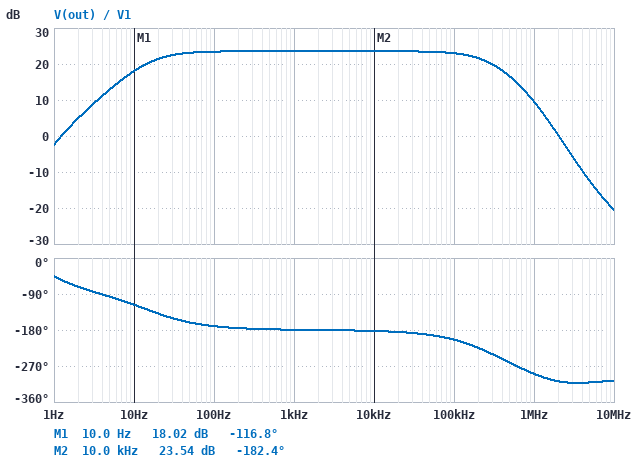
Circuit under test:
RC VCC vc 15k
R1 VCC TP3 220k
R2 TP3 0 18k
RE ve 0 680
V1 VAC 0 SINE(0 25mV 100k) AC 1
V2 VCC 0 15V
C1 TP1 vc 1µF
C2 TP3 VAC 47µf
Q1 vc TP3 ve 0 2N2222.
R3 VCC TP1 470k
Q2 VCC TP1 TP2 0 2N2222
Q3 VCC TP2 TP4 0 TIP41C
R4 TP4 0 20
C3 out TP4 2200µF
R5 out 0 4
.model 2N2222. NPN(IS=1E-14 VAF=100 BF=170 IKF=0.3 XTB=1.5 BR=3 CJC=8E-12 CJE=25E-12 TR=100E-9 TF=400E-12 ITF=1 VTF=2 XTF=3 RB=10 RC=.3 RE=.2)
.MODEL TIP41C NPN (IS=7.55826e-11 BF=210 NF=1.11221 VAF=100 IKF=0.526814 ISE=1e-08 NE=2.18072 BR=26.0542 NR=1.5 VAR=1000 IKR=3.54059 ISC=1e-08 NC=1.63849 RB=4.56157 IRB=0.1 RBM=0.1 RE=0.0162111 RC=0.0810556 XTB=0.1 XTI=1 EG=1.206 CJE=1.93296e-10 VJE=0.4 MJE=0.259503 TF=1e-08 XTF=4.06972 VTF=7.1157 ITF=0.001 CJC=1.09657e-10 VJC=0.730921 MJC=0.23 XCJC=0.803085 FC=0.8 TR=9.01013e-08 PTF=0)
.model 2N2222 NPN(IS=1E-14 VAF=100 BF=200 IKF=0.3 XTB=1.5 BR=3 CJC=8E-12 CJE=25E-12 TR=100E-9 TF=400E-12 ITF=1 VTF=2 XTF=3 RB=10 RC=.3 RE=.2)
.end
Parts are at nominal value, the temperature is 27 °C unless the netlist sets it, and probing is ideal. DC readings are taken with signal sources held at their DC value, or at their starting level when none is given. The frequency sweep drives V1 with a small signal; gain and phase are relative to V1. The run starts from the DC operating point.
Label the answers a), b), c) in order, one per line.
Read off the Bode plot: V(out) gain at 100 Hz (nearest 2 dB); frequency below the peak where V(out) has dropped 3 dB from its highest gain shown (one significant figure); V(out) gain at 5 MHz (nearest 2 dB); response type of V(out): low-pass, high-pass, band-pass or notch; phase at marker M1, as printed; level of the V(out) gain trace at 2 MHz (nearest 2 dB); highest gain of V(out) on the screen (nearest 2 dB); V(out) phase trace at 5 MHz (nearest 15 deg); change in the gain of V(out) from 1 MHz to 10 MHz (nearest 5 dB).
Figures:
a) 24 dB
b) 20 Hz
c) -12 dB
d) band-pass
e) -116.8 deg
f) 0 dB
g) 24 dB
h) -315 deg
i) -30 dB
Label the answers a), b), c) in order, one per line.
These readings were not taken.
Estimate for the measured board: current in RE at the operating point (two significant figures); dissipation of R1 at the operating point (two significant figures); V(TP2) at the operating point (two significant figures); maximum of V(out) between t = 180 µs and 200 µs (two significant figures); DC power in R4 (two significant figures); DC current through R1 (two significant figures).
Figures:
a) 640 µA
b) 880 µW
c) 7.2 V
d) 350 mV
e) 2.1 W
f) 63 µA
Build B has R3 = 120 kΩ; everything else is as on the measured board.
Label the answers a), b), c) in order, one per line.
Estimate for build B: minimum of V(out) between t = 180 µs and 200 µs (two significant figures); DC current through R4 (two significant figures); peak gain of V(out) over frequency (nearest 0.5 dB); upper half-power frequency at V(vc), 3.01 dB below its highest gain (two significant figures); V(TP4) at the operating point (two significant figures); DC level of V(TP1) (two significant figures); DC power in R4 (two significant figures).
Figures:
a) -310 mV
b) 510 mA
c) 22.5 dB
d) 67 kHz
e) 10 V
f) 12 V
g) 5.2 W
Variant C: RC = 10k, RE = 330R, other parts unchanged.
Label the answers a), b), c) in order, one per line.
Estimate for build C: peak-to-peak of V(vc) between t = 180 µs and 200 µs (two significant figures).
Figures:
a) 1.2 V
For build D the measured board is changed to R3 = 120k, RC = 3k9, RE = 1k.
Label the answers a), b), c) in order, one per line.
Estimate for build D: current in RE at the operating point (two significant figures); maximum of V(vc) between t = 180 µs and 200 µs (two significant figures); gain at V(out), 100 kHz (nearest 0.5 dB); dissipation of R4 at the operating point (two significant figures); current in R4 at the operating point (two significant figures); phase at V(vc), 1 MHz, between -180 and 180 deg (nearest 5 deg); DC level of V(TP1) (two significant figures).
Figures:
a) 460 µA
b) 13 V
c) 9.5 dB
d) 5.2 W
e) 510 mA
f) 125 deg
g) 12 V
